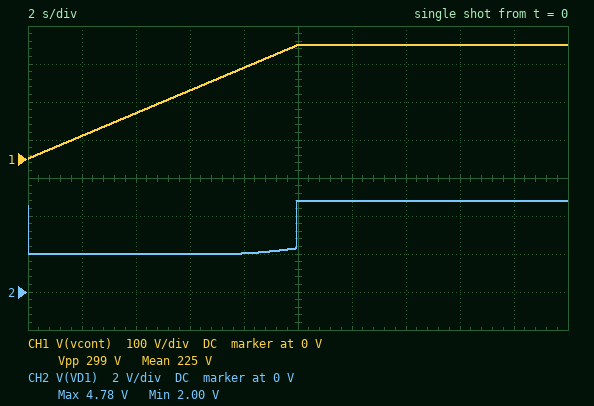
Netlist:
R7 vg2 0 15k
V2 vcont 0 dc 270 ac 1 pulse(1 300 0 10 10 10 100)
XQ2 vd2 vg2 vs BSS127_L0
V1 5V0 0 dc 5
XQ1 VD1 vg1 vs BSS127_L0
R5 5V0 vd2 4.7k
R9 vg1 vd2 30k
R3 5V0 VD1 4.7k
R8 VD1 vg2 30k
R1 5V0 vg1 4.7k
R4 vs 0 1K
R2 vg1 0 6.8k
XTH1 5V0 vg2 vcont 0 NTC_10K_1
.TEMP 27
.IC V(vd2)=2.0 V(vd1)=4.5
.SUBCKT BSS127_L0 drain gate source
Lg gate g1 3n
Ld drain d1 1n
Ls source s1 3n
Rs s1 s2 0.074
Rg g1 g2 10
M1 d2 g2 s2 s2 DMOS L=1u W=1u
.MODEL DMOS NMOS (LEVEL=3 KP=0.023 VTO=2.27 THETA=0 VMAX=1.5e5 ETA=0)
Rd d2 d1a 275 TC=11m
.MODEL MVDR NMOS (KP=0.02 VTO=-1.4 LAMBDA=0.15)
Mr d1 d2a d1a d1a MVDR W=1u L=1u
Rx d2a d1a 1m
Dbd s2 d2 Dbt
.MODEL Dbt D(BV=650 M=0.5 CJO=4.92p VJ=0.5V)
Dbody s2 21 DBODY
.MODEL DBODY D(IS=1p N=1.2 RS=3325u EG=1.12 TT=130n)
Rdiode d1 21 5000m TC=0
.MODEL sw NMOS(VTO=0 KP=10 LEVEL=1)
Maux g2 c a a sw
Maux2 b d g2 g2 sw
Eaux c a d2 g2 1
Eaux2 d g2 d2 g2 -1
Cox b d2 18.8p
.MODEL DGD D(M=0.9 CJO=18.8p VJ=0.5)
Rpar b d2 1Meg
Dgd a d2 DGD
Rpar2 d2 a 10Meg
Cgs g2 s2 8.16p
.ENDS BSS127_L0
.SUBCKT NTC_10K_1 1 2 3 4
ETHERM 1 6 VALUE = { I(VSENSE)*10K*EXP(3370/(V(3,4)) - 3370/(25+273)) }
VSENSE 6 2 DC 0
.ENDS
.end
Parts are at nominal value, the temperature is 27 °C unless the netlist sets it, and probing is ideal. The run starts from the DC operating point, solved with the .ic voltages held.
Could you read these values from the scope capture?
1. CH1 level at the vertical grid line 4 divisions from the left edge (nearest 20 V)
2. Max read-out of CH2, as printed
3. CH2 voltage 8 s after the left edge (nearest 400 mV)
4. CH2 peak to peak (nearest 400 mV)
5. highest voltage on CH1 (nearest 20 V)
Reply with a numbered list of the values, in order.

1. 240 V
2. 4.78 V
3. 2.0 V
4. 2.8 V
5. 300 V
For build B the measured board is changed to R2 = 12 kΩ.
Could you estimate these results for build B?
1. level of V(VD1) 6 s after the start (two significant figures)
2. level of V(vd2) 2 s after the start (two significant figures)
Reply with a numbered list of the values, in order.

1. 1.1 V
2. 4.8 V
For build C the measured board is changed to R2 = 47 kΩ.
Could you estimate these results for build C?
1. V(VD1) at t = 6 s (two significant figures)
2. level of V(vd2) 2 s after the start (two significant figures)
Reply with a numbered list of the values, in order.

1. 1.1 V
2. 4.9 V
